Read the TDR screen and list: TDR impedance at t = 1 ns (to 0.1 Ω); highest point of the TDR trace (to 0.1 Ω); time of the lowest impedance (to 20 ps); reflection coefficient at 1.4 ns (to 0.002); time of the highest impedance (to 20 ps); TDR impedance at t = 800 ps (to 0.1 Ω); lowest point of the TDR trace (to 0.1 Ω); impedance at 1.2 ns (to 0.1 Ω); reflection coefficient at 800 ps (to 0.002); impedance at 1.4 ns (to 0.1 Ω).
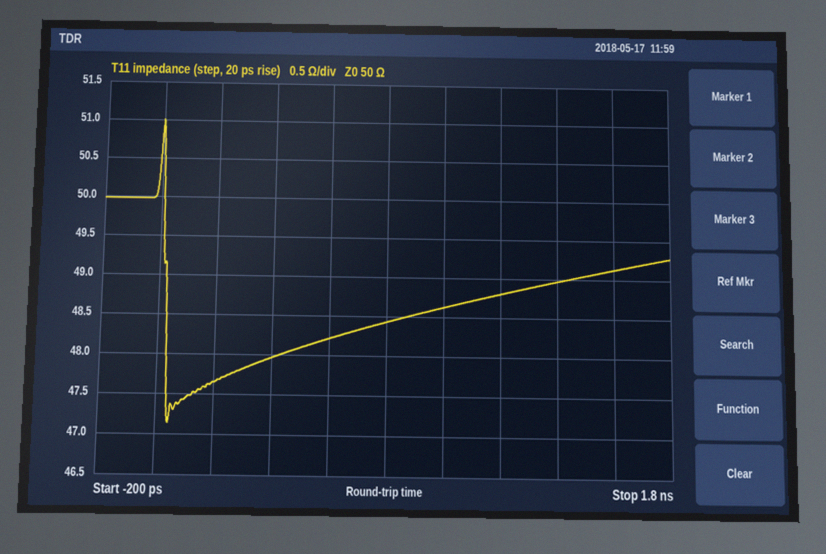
48.6 Ω
51.0 Ω
40 ps
-0.010
0 ps
48.4 Ω
47.1 Ω
48.8 Ω
-0.016
49.0 Ω
